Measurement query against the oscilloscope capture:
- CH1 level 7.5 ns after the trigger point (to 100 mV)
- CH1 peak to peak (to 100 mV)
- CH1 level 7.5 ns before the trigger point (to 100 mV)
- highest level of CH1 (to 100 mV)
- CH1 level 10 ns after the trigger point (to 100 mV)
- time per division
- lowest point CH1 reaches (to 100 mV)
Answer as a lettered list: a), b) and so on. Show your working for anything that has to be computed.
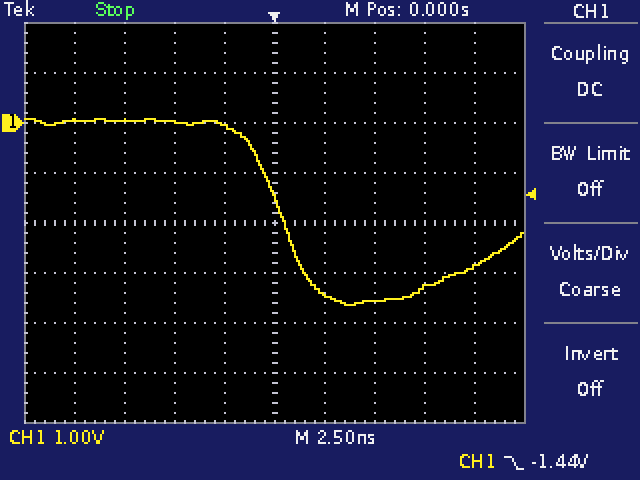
a) -3.3 V
b) 100 mV − (-3.6 V) = 3.7 V
c) 100 mV
d) 100 mV
e) -2.9 V
f) 2.5 ns
g) -3.6 V
